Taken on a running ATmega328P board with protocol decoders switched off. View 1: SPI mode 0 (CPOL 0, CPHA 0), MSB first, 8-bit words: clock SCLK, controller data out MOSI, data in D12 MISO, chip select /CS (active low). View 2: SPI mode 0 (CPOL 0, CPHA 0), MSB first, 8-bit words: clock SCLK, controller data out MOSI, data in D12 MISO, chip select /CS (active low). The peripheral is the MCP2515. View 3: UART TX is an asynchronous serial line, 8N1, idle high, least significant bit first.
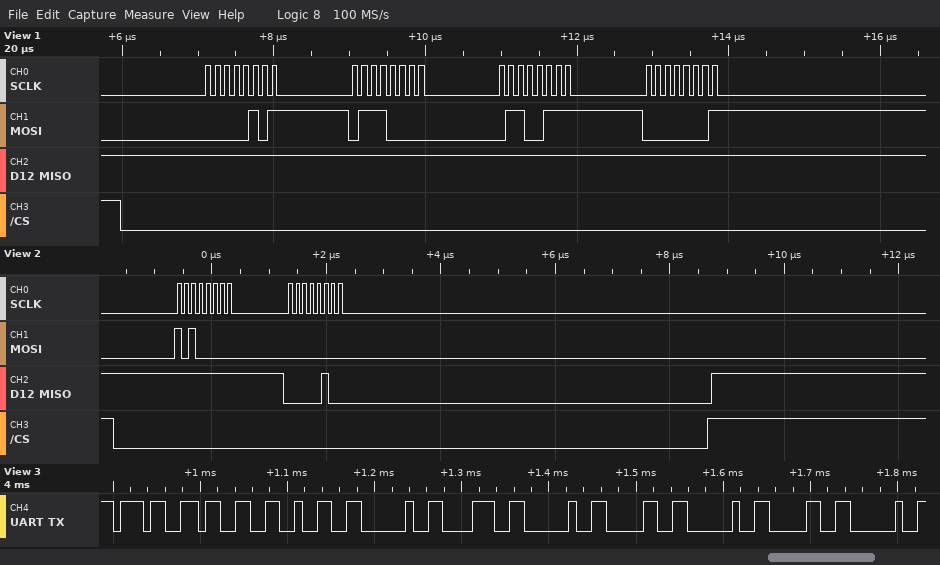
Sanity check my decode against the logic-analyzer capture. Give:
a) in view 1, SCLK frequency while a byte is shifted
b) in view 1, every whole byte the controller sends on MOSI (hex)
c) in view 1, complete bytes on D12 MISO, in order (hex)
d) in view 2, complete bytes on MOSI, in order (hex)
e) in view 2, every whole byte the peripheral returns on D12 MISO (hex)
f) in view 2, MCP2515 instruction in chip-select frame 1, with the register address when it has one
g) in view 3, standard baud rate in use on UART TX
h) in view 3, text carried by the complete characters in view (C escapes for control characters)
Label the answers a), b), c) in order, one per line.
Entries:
a) 8 MHz
b) 05 70 67 01
c) FF FF FF FF
d) A0 00
e) FF 04
f) READ STATUS
g) 115200 baud
h) "732 8 0 0 "
